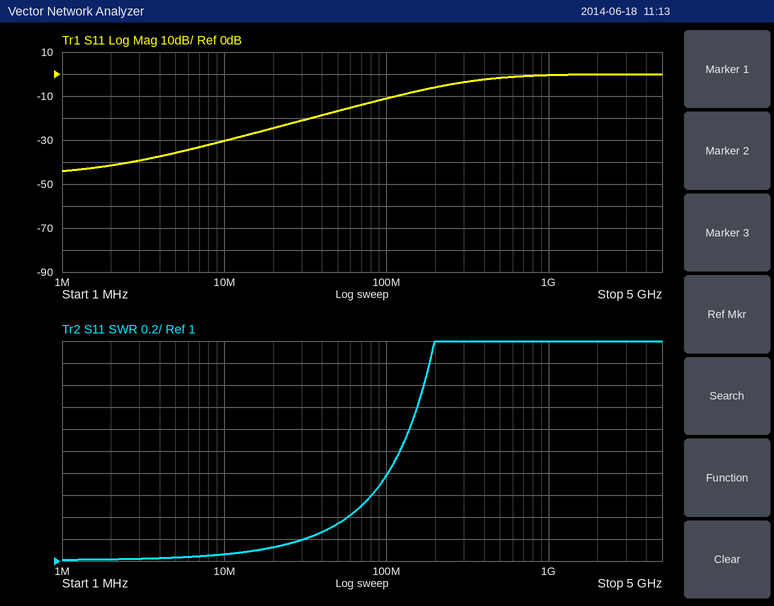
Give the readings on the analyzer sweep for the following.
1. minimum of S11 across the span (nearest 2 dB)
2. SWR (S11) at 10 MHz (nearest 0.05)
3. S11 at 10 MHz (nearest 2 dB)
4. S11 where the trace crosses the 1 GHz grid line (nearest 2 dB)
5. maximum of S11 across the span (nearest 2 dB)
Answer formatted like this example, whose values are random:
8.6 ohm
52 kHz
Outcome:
-44 dB
1.05
-30 dB
0 dB
0 dB
